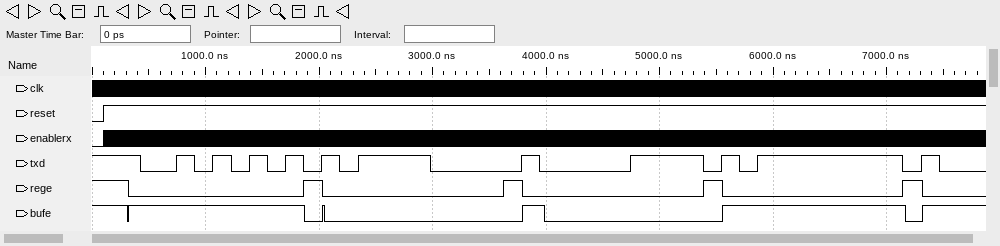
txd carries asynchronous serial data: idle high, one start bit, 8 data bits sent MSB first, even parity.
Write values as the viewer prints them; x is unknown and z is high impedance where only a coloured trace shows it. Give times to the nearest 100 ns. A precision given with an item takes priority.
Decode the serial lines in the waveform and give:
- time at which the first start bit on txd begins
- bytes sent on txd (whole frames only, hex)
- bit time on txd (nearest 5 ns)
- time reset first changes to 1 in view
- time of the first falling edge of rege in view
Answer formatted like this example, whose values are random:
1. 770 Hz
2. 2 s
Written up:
1. 400 ns
2. 55, F0, 0F, FF
3. 160 ns
4. 100 ns
5. 300 ns
